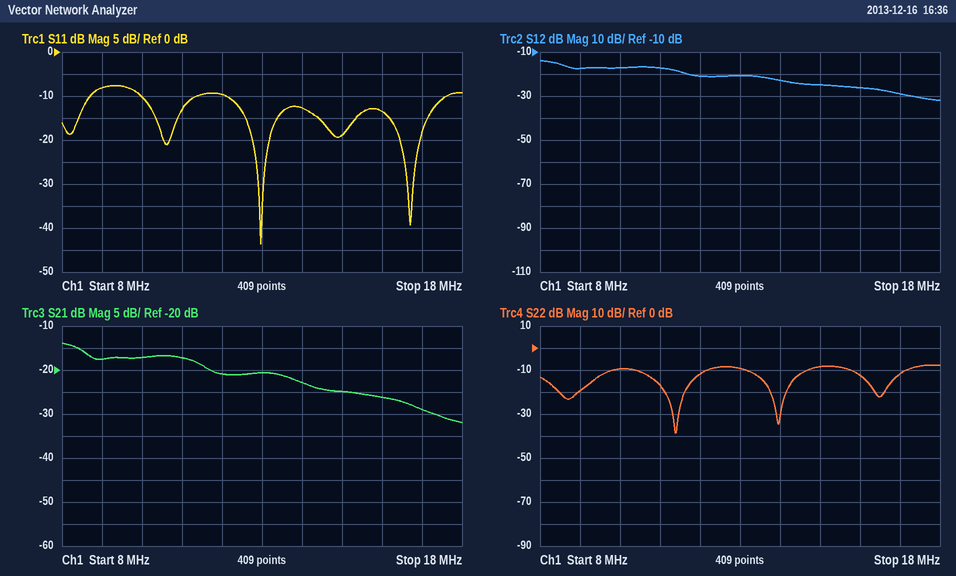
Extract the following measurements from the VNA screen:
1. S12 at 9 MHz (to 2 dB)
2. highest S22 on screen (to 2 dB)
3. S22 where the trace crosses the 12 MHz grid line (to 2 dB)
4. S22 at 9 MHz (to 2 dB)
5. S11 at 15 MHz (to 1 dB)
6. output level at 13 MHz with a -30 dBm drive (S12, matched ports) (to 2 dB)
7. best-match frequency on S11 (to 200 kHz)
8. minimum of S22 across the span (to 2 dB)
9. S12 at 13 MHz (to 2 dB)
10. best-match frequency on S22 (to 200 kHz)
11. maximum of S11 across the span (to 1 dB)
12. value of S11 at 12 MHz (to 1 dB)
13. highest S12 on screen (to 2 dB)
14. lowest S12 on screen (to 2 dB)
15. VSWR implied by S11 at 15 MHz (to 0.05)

-18 dB
-8 dB
-12 dB
-20 dB
-19 dB
-50 dBm
13.0 MHz
-38 dB
-20 dB
11.4 MHz
-8 dB
-10 dB
-14 dB
-32 dB
1.25
